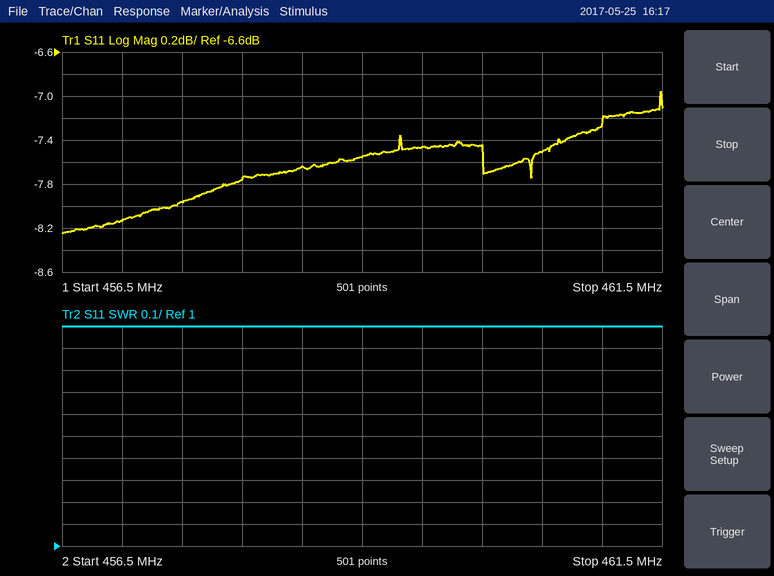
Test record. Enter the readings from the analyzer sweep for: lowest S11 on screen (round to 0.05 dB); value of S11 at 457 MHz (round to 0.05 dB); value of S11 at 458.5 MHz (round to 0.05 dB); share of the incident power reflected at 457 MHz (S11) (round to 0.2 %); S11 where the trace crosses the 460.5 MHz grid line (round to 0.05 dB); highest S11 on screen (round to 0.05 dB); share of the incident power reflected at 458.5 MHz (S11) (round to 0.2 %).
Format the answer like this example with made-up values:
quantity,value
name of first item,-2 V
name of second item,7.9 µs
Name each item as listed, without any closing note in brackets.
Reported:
quantity,value
lowest S11 on screen,-8.25 dB
value of S11 at 457 MHz,-8.15 dB
value of S11 at 458.5 MHz,-7.65 dB
share of the incident power reflected at 457 MHz (S11),15.4 %
S11 where the trace crosses the 460.5 MHz grid line,-7.50 dB
highest S11 on screen,-6.95 dB
share of the incident power reflected at 458.5 MHz (S11),17.2 %
